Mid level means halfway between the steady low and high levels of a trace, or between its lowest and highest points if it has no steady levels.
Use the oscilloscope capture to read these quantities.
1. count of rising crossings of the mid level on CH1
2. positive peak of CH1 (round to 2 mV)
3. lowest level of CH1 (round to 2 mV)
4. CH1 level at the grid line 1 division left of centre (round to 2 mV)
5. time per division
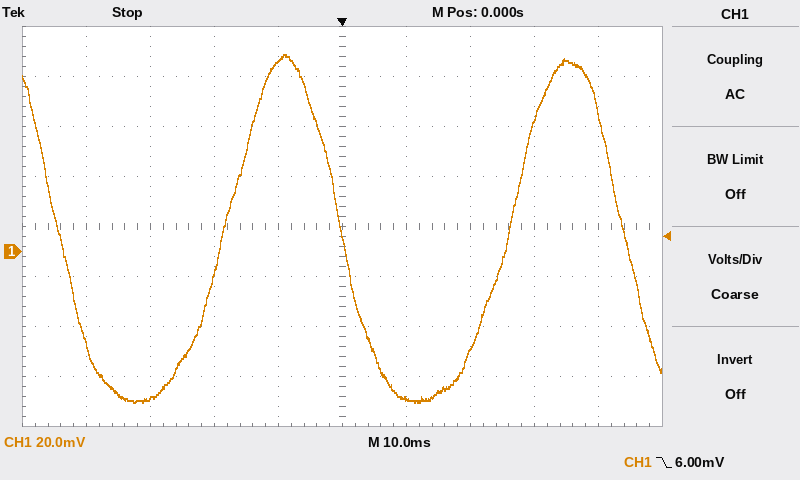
2
78 mV
-60 mV
76 mV
10 ms
